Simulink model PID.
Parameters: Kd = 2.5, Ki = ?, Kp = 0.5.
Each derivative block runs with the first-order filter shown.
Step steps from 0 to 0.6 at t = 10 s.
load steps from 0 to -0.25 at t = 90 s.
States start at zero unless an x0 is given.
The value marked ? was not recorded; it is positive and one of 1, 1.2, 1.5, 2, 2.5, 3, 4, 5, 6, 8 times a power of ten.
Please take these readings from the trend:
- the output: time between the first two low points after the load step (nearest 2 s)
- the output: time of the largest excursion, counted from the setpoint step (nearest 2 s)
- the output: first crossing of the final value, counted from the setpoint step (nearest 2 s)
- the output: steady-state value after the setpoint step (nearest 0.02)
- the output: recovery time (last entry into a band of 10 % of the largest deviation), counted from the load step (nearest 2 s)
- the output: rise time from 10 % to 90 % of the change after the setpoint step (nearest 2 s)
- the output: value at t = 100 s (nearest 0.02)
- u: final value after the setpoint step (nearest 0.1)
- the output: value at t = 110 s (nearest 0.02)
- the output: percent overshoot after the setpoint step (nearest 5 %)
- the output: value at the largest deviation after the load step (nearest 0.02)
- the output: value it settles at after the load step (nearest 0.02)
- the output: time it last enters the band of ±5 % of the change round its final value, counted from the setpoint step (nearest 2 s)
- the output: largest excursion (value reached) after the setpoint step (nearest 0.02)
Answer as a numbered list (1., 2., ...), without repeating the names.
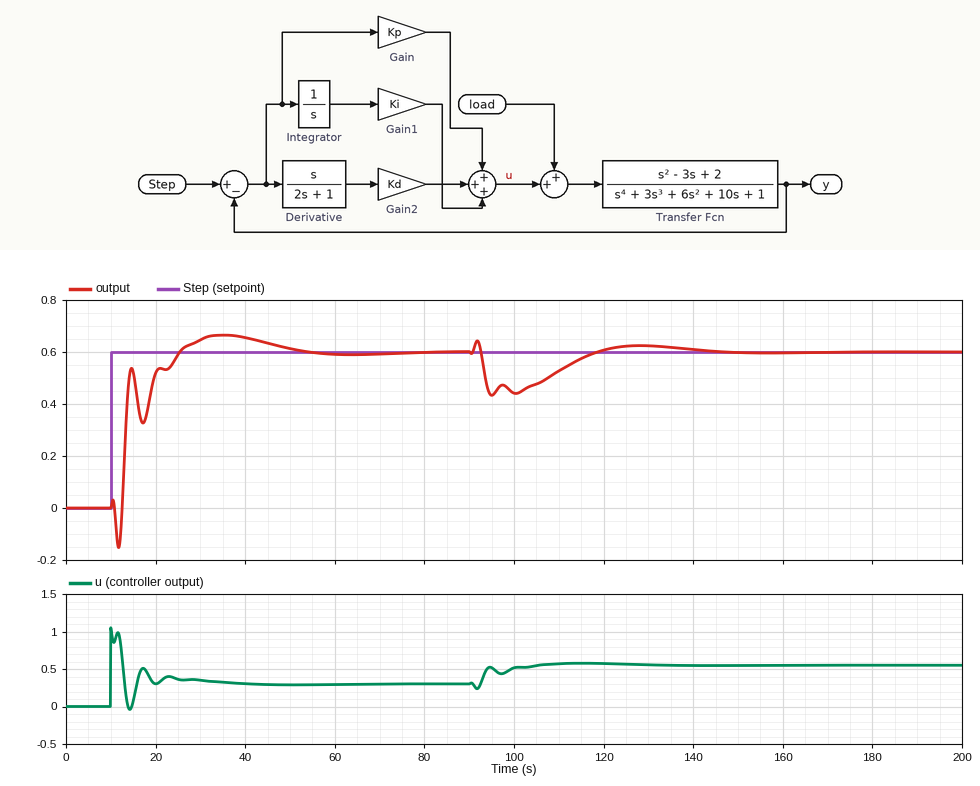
1. 6 s
2. 26 s
3. 16 s
4. 0.60
5. 46 s
6. 10 s
7. 0.44
8. 0.3
9. 0.52
10. 10 %
11. 0.44
12. 0.60
13. 36 s
14. 0.66
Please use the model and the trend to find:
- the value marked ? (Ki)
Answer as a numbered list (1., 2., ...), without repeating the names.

1. 0.12
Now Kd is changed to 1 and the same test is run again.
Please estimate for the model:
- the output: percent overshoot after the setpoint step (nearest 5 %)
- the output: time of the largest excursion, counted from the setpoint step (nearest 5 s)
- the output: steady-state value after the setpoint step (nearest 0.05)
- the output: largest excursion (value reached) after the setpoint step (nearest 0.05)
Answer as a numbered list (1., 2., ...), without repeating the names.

1. 15 %
2. 20 s
3. 0.60
4. 0.70
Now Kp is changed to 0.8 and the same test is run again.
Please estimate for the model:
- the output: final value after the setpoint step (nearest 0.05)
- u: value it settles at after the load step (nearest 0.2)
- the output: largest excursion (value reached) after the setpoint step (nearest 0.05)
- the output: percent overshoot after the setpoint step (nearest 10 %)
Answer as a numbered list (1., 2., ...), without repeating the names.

1. 0.60
2. 0.6
3. 0.70
4. 20 %
